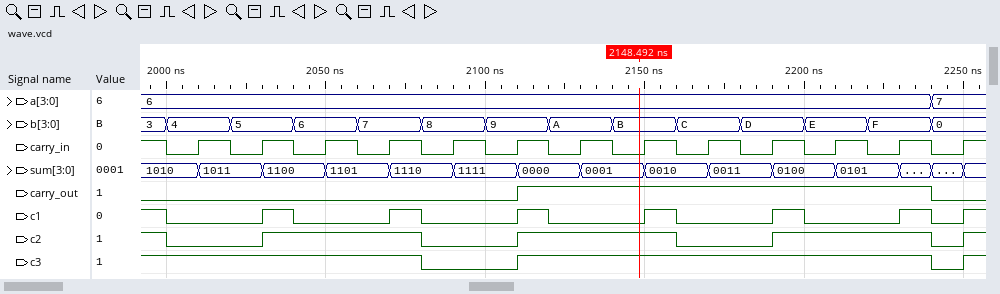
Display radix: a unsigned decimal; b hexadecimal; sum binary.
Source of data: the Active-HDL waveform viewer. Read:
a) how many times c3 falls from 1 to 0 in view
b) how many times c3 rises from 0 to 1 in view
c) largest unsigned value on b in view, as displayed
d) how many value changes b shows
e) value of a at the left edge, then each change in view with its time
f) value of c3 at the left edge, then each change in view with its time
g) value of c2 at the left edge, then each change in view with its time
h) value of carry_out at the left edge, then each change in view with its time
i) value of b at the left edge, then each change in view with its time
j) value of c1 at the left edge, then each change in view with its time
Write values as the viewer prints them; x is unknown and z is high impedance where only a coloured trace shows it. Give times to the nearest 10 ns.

2
2
F
13
6, 7 at 2240 ns
1, 0 at 2080 ns, 1 at 2110 ns, 0 at 2240 ns, 1 at 2250 ns
1, 0 at 2000 ns, 1 at 2030 ns, 0 at 2080 ns, 1 at 2110 ns, 0 at 2160 ns, 1 at 2190 ns, 0 at 2240 ns, 1 at 2250 ns
0, 1 at 2110 ns, 0 at 2240 ns
3, 4 at 2000 ns, 5 at 2020 ns, 6 at 2040 ns, 7 at 2060 ns, 8 at 2080 ns, 9 at 2100 ns, A at 2120 ns, B at 2140 ns, C at 2160 ns, D at 2180 ns, E at 2200 ns, F at 2220 ns, 0 at 2240 ns
1, 0 at 2000 ns, 1 at 2030 ns, 0 at 2040 ns, 1 at 2070 ns, 0 at 2080 ns, 1 at 2110 ns, 0 at 2120 ns, 1 at 2150 ns, 0 at 2160 ns, 1 at 2190 ns, 0 at 2200 ns, 1 at 2230 ns, 0 at 2240 ns, 1 at 2250 ns
